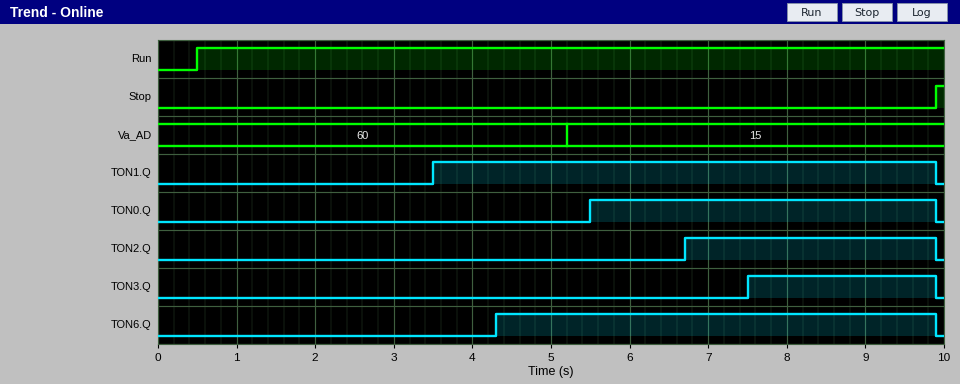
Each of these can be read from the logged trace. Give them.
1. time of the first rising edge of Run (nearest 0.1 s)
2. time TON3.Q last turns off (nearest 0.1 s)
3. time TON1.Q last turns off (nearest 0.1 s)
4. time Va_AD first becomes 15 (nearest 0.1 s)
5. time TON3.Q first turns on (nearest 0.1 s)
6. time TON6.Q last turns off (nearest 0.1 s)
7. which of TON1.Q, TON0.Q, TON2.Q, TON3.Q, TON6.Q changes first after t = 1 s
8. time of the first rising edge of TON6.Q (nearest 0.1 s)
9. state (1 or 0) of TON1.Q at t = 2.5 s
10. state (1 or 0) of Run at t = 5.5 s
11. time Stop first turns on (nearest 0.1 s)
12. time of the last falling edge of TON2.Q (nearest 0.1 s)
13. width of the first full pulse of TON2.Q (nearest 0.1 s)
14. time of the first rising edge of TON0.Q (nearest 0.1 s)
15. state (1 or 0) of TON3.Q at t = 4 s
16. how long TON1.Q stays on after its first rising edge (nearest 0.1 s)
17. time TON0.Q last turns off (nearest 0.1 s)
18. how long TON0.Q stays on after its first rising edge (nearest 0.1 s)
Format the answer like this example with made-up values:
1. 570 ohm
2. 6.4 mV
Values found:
1. 0.5 s
2. 9.9 s
3. 9.9 s
4. 5.2 s
5. 7.5 s
6. 9.9 s
7. TON1.Q
8. 4.3 s
9. 0
10. 1
11. 9.9 s
12. 9.9 s
13. 3.2 s
14. 5.5 s
15. 0
16. 6.4 s
17. 9.9 s
18. 4.4 s
